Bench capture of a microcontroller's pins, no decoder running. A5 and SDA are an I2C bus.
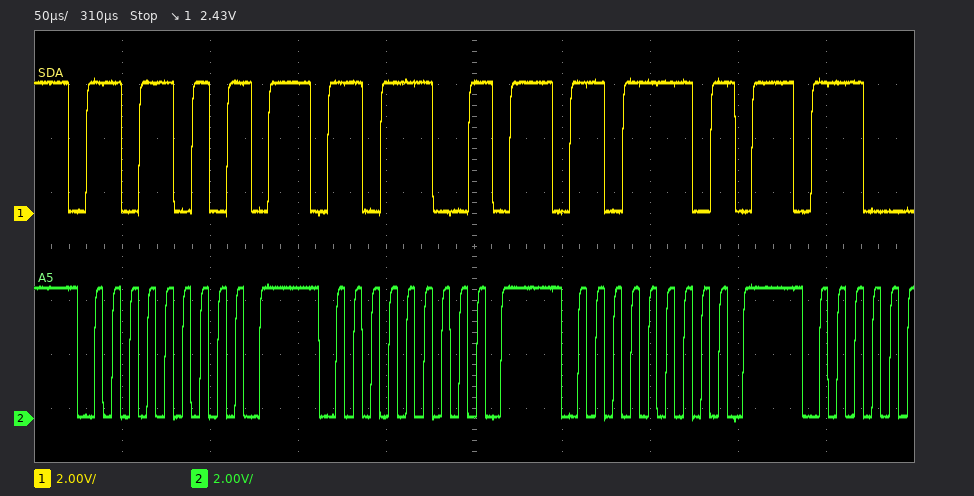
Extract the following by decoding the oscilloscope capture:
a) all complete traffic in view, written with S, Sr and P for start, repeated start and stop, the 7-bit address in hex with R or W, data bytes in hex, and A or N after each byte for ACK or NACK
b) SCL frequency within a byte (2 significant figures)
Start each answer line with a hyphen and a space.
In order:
- S 6DW N P S 6EW N P S 6FW N P
- 100 kHz
